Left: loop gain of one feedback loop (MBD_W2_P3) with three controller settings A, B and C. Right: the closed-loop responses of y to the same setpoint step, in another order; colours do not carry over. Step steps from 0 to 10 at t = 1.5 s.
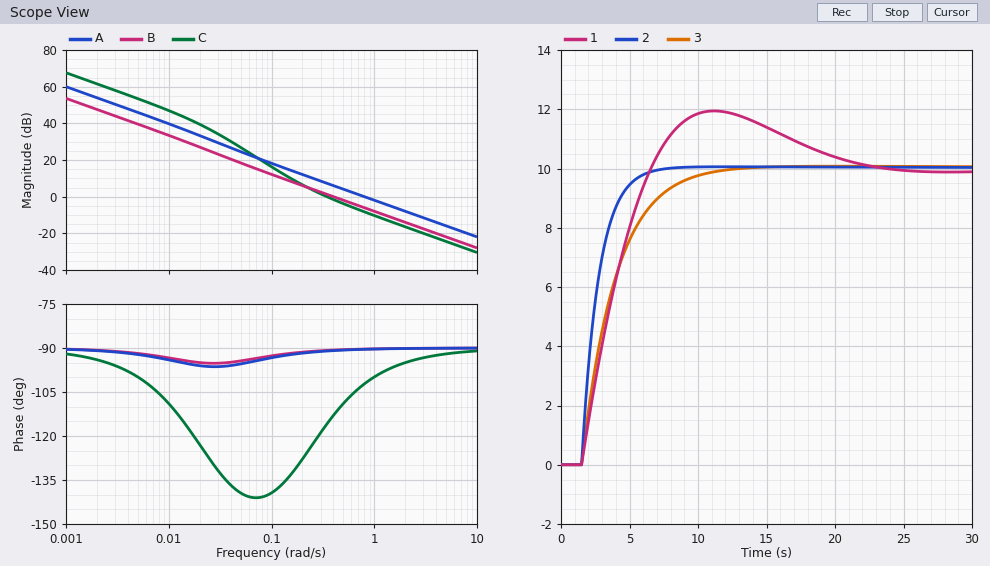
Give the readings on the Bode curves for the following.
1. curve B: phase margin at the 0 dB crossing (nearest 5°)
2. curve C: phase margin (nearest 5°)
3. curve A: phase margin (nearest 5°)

90°
65°
90°
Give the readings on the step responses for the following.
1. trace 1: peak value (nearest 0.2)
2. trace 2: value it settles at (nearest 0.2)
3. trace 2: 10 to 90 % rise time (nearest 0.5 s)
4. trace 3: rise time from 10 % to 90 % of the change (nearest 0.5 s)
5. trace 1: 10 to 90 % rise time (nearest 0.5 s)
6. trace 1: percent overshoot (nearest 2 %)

12.0
10.0
2.5 s
5.5 s
4.0 s
20 %
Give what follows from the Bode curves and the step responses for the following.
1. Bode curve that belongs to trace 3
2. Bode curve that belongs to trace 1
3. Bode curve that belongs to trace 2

B
C
A
